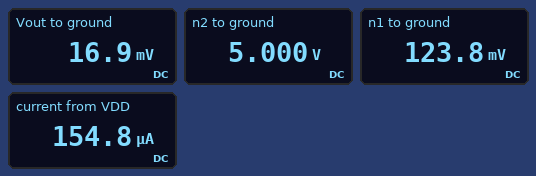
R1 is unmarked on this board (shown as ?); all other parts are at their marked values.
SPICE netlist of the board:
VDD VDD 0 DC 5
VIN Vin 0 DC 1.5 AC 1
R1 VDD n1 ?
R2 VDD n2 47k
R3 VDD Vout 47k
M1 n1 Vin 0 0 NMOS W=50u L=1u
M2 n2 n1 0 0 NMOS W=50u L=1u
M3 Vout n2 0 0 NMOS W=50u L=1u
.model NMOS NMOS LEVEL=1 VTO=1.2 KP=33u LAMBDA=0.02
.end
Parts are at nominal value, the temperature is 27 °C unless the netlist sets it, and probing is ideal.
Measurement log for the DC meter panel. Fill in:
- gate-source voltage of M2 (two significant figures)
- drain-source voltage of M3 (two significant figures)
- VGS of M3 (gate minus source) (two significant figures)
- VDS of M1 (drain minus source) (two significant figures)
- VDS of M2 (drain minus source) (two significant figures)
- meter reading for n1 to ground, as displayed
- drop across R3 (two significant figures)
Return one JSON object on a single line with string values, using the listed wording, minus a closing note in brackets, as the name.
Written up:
{"gate-source voltage of M2": "120 mV", "drain-source voltage of M3": "17 mV", "VGS of M3 (gate minus source)": "5.0 V", "VDS of M1 (drain minus source)": "120 mV", "VDS of M2 (drain minus source)": "5.0 V", "meter reading for n1 to ground, as displayed": "123.8 mV", "drop across R3": "5.0 V"}
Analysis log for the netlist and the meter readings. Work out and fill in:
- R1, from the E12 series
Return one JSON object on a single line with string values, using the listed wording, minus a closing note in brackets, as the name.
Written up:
{"R1, from the E12 series": "100 kΩ"}
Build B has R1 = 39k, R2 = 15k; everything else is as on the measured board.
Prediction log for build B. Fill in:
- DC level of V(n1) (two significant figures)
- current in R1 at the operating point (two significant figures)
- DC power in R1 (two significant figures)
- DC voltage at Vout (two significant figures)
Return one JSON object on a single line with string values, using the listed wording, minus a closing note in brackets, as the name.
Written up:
{"DC level of V(n1)": "2.0 V", "current in R1 at the operating point": "77 µA", "DC power in R1": "230 µW", "DC voltage at Vout": "5.0 V"}
